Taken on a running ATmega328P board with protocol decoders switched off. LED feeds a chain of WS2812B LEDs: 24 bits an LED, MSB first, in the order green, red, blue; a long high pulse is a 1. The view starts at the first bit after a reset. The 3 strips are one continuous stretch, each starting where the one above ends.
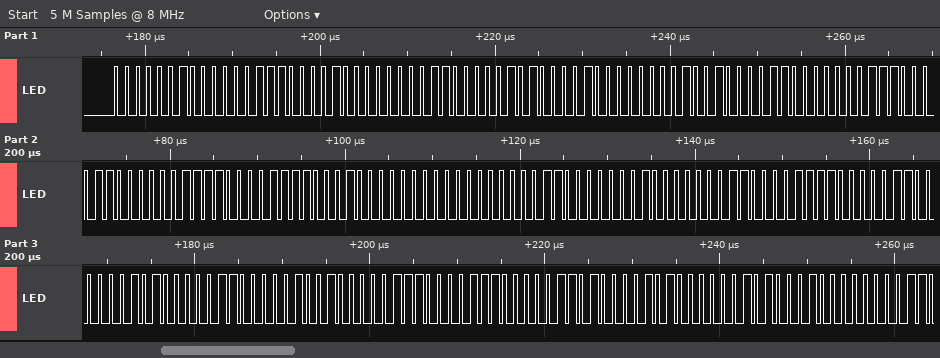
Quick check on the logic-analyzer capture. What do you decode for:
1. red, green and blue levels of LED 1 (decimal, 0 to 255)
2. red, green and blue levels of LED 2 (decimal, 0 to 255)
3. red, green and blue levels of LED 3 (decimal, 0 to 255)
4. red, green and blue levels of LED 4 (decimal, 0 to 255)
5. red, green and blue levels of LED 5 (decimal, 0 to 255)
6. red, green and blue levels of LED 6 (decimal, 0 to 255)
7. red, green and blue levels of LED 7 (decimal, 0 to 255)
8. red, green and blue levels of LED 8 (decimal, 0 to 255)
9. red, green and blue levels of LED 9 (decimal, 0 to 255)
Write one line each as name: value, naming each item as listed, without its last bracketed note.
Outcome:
red, green and blue levels of LED 1: 7, 2, 8
red, green and blue levels of LED 2: 10, 6, 16
red, green and blue levels of LED 3: 12, 9, 7
red, green and blue levels of LED 4: 15, 12, 15
red, green and blue levels of LED 5: 0, 16, 6
red, green and blue levels of LED 6: 3, 2, 15
red, green and blue levels of LED 7: 5, 6, 6
red, green and blue levels of LED 8: 7, 9, 14
red, green and blue levels of LED 9: 10, 13, 5
